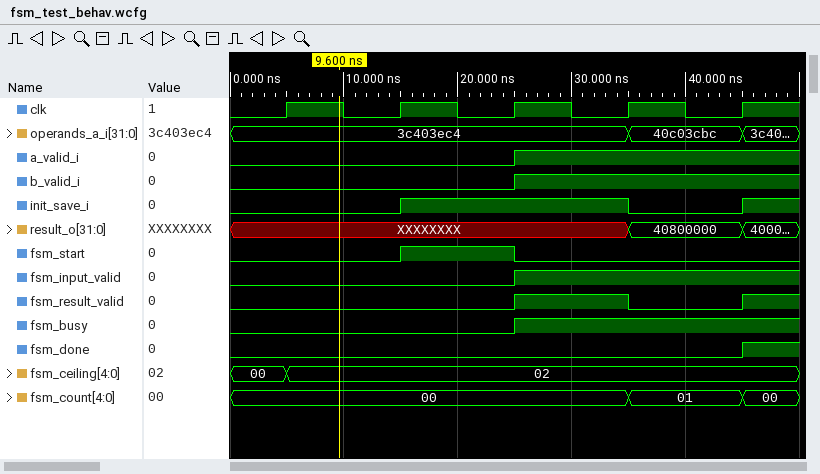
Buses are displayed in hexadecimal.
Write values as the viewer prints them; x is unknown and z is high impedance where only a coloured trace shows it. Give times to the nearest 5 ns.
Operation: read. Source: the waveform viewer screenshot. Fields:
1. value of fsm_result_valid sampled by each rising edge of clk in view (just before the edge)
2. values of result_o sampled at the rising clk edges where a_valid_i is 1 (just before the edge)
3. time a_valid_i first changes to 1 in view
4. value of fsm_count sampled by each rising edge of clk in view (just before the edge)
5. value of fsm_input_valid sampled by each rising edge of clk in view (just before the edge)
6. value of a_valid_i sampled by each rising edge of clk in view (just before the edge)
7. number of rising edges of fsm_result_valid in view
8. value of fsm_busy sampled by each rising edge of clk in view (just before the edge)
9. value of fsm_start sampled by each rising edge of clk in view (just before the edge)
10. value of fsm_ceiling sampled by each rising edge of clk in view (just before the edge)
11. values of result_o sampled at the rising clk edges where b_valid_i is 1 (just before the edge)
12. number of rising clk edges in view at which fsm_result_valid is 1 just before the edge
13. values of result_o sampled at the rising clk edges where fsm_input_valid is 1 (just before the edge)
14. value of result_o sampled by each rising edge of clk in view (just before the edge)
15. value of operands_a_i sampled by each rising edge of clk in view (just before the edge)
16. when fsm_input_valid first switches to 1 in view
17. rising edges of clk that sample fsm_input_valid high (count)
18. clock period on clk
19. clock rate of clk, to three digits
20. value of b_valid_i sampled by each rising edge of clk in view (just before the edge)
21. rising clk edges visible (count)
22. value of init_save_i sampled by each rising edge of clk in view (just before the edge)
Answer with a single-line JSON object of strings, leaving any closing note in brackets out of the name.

{"value of fsm_result_valid sampled by each rising edge of clk in view": "0 0 0 1 0", "values of result_o sampled at the rising clk edges where a_valid_i is 1": "XXXXXXXX, 40800000", "time a_valid_i first changes to 1 in view": "25 ns", "value of fsm_count sampled by each rising edge of clk in view": "00, 00, 00, 00, 01", "value of fsm_input_valid sampled by each rising edge of clk in view": "0 0 0 1 1", "value of a_valid_i sampled by each rising edge of clk in view": "0 0 0 1 1", "number of rising edges of fsm_result_valid in view": "2", "value of fsm_busy sampled by each rising edge of clk in view": "0 0 0 1 1", "value of fsm_start sampled by each rising edge of clk in view": "0 0 1 0 0", "value of fsm_ceiling sampled by each rising edge of clk in view": "00, 02, 02, 02, 02", "values of result_o sampled at the rising clk edges where b_valid_i is 1": "XXXXXXXX, 40800000", "number of rising clk edges in view at which fsm_result_valid is 1 just before the edge": "1", "values of result_o sampled at the rising clk edges where fsm_input_valid is 1": "XXXXXXXX, 40800000", "value of result_o sampled by each rising edge of clk in view": "XXXXXXXX, XXXXXXXX, XXXXXXXX, XXXXXXXX, 40800000", "value of operands_a_i sampled by each rising edge of clk in view": "3c403ec4, 3c403ec4, 3c403ec4, 3c403ec4, 40c03cbc", "when fsm_input_valid first switches to 1 in view": "25 ns", "rising edges of clk that sample fsm_input_valid high": "2", "clock period on clk": "10 ns", "clock rate of clk, to three digits": "100 MHz", "value of b_valid_i sampled by each rising edge of clk in view": "0 0 0 1 1", "rising clk edges visible": "5", "value of init_save_i sampled by each rising edge of clk in view": "0 0 1 1 0"}
